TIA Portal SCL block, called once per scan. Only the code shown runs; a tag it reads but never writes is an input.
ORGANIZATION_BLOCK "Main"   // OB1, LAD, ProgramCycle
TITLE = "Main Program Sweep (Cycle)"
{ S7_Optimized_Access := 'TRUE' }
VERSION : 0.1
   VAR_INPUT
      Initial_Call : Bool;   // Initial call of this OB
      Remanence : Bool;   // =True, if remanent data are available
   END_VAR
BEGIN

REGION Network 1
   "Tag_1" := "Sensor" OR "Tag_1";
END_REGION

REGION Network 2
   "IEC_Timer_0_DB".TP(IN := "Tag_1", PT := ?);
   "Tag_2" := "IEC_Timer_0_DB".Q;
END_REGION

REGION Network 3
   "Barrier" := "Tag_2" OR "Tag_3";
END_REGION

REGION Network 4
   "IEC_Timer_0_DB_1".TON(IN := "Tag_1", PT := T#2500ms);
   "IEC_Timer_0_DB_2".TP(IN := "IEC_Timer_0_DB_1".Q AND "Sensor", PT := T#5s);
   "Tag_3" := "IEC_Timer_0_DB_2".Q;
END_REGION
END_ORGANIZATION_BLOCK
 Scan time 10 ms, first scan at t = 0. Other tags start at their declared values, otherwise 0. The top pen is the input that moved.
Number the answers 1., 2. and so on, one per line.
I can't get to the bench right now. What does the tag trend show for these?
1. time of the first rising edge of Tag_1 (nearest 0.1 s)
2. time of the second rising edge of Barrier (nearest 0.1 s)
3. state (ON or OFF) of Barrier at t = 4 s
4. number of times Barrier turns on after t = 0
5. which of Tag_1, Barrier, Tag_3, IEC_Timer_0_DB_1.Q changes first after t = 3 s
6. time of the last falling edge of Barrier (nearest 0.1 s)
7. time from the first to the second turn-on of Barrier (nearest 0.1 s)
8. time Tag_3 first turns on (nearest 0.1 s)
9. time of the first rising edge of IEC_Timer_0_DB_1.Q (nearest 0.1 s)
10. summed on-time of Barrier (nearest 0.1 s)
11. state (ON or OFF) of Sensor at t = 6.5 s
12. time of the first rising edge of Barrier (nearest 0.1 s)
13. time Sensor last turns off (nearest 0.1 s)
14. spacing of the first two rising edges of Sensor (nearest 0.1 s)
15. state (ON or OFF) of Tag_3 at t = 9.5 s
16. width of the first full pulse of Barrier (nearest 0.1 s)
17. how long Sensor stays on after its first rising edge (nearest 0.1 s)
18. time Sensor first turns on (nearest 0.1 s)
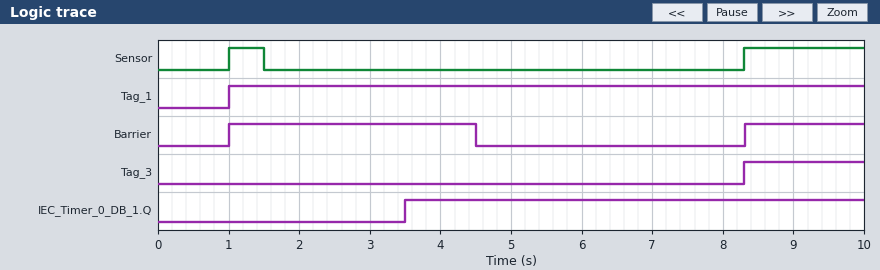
1. 1.0 s
2. 8.3 s
3. ON
4. 2
5. IEC_Timer_0_DB_1.Q
6. 4.5 s
7. 7.3 s
8. 8.3 s
9. 3.5 s
10. 5.2 s
11. OFF
12. 1.0 s
13. 1.5 s
14. 7.3 s
15. ON
16. 3.5 s
17. 0.5 s
18. 1.0 s
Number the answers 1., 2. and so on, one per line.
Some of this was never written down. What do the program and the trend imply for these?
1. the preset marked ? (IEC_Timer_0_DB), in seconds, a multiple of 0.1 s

1. 3.5 s
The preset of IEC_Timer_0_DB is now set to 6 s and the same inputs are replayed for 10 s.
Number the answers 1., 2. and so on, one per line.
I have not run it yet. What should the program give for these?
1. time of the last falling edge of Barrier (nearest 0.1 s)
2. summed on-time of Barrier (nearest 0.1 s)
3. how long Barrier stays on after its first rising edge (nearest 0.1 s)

1. 7.0 s
2. 7.7 s
3. 6.0 s
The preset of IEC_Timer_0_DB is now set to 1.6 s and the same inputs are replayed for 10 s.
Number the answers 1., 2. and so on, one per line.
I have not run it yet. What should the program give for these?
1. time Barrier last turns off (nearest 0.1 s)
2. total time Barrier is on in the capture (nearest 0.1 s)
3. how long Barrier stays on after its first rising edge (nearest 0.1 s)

1. 2.6 s
2. 3.3 s
3. 1.6 s
